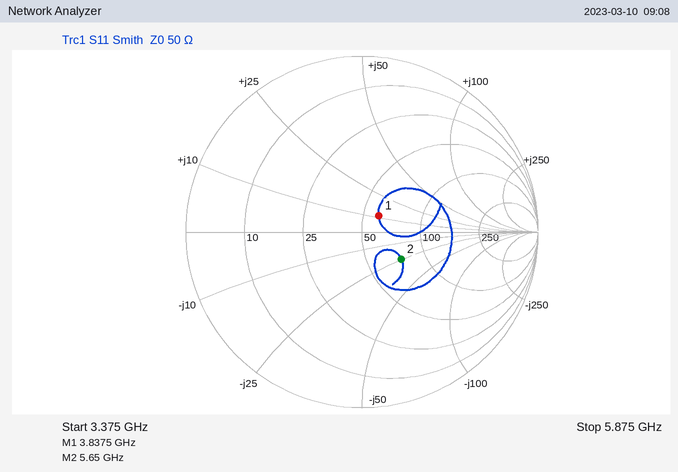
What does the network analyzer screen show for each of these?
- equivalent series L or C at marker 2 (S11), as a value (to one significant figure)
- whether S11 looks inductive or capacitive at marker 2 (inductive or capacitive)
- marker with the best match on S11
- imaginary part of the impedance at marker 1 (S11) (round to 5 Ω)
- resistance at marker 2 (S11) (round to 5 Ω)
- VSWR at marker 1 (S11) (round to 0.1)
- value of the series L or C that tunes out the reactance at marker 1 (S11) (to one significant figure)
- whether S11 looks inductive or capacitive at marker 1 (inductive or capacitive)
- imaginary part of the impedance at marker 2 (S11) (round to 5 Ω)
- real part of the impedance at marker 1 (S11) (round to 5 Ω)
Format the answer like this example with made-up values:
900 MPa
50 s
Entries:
1 pF
capacitive
marker 1
+10 Ω
75 Ω
1.3
4 pF
inductive
-25 Ω
60 Ω
